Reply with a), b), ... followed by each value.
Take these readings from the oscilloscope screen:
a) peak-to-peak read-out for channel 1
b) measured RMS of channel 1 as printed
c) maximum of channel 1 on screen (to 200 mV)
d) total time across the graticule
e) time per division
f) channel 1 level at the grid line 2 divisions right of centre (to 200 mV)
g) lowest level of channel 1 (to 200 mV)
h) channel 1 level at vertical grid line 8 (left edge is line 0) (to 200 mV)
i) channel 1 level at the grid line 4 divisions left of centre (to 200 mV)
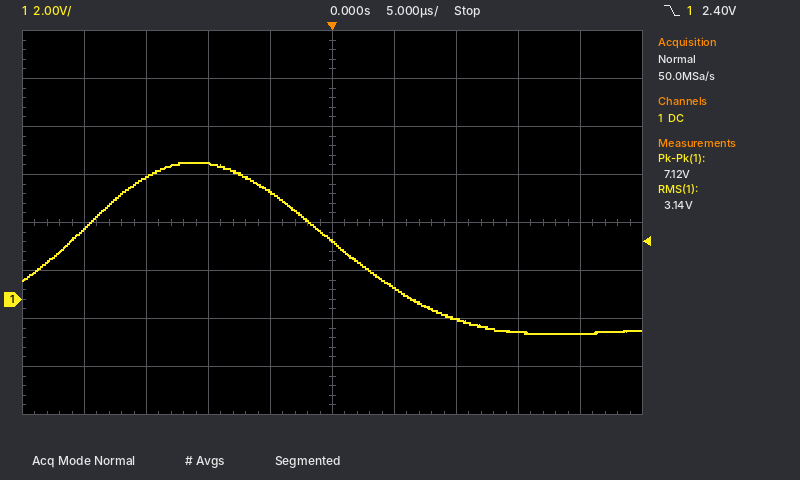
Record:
a) 7.12 V
b) 3.14 V
c) 5.6 V
d) 50 µs
e) 5 µs
f) -800 mV
g) -1.4 V
h) -1.4 V
i) 3.0 V
